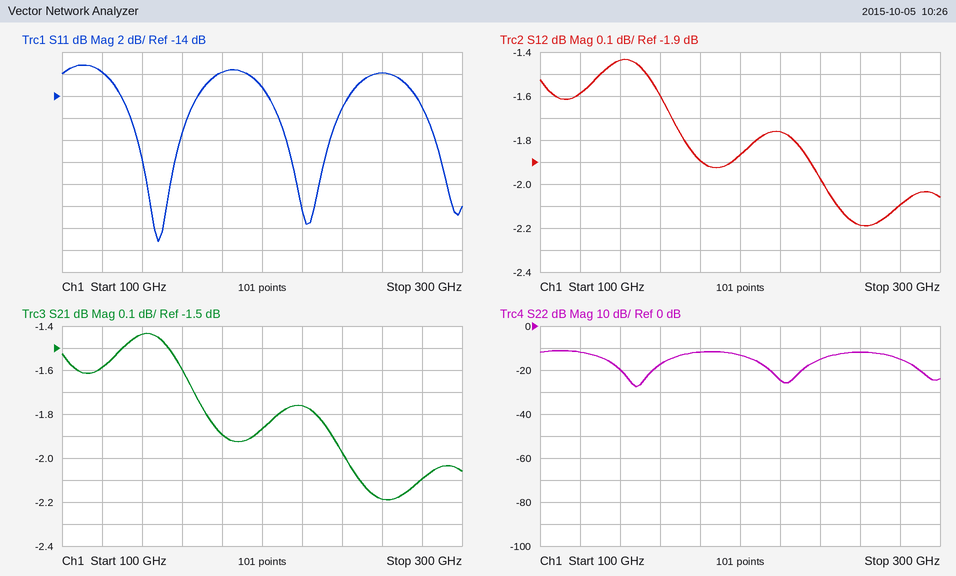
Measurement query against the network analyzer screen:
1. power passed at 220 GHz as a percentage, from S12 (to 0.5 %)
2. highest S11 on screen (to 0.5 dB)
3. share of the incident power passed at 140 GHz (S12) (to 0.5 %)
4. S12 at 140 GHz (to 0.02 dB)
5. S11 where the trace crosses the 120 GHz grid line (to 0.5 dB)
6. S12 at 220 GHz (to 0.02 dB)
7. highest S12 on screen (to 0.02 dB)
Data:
66.5 %
-11.0 dB
72.0 %
-1.44 dB
-12.0 dB
-1.76 dB
-1.44 dB
